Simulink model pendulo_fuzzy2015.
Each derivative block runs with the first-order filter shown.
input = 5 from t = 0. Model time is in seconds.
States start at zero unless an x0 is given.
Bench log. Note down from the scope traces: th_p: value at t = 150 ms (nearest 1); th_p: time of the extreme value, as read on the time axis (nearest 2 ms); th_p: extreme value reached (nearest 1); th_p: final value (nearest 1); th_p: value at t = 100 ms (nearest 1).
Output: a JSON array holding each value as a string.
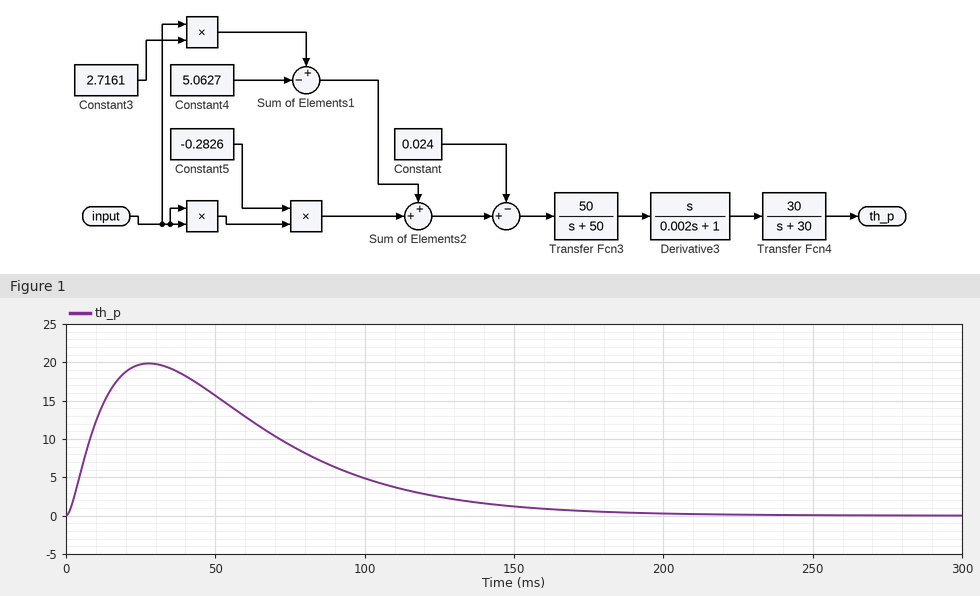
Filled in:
["1", "28 ms", "20", "0", "5"]
